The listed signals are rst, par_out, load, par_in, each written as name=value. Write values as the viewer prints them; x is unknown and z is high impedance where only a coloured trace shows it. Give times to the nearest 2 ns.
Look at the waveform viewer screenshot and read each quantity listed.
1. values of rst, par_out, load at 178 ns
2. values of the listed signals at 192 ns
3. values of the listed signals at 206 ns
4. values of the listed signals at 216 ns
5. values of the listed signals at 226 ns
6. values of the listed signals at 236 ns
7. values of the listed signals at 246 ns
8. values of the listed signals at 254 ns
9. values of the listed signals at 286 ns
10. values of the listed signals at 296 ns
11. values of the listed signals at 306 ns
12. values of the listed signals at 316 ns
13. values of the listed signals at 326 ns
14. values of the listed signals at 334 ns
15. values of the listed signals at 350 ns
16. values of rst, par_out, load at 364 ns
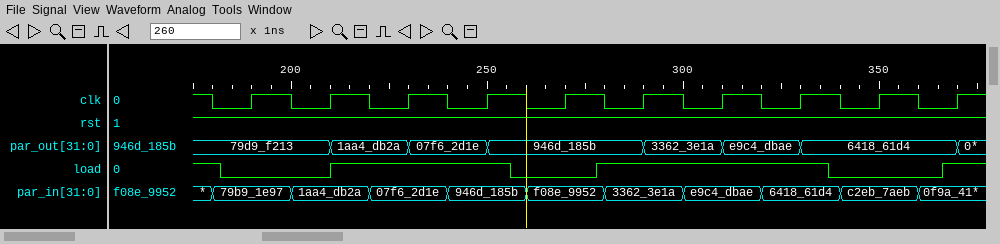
rst=1, par_out=79d9_f213, load=1
rst=1, par_out=79d9_f213, load=0, par_in=79b9_1e97
rst=1, par_out=79d9_f213, load=0, par_in=1aa4_db2a
rst=1, par_out=1aa4_db2a, load=1, par_in=1aa4_db2a
rst=1, par_out=1aa4_db2a, load=1, par_in=07f6_2d1e
rst=1, par_out=07f6_2d1e, load=1, par_in=07f6_2d1e
rst=1, par_out=07f6_2d1e, load=1, par_in=946d_185b
rst=1, par_out=946d_185b, load=1, par_in=946d_185b
rst=1, par_out=946d_185b, load=1, par_in=3362_3e1a
rst=1, par_out=3362_3e1a, load=1, par_in=3362_3e1a
rst=1, par_out=3362_3e1a, load=1, par_in=e9c4_dbae
rst=1, par_out=e9c4_dbae, load=1, par_in=e9c4_dbae
rst=1, par_out=e9c4_dbae, load=1, par_in=6418_61d4
rst=1, par_out=6418_61d4, load=1, par_in=6418_61d4
rst=1, par_out=6418_61d4, load=0, par_in=c2eb_7aeb
rst=1, par_out=6418_61d4, load=0
